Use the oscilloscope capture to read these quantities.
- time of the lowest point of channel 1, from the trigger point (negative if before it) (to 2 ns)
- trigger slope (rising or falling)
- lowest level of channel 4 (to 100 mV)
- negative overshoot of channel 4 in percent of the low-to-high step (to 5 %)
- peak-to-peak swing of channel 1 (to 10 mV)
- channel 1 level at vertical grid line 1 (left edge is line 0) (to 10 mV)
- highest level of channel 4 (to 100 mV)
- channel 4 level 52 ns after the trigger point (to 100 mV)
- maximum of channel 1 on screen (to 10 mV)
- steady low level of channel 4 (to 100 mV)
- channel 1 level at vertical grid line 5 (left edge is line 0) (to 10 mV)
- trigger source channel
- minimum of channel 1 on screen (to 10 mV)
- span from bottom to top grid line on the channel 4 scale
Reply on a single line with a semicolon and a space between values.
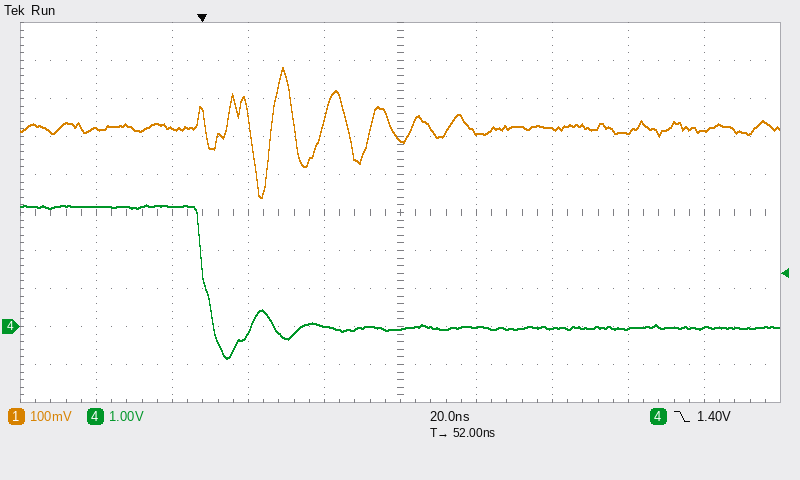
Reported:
+16 ns; falling; -800 mV; 25 %; 340 mV; 520 mV; 3.2 V; -100 mV; 680 mV; 0.0 V; 490 mV; channel 4; 340 mV; 10 V
